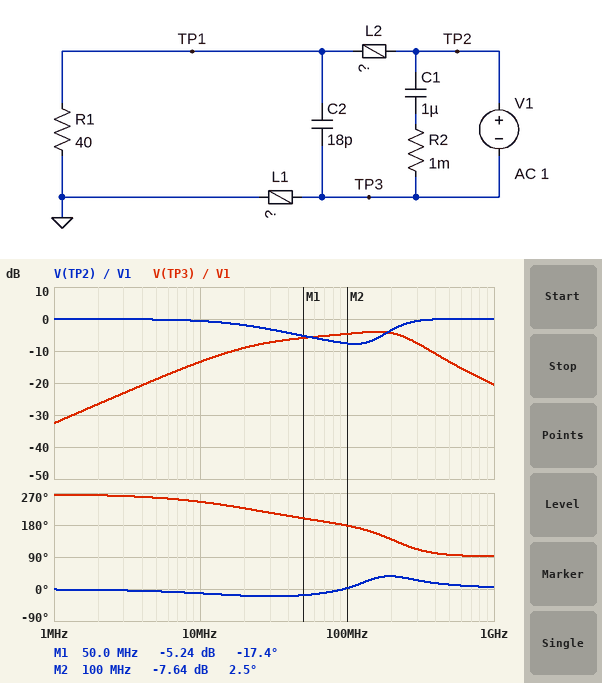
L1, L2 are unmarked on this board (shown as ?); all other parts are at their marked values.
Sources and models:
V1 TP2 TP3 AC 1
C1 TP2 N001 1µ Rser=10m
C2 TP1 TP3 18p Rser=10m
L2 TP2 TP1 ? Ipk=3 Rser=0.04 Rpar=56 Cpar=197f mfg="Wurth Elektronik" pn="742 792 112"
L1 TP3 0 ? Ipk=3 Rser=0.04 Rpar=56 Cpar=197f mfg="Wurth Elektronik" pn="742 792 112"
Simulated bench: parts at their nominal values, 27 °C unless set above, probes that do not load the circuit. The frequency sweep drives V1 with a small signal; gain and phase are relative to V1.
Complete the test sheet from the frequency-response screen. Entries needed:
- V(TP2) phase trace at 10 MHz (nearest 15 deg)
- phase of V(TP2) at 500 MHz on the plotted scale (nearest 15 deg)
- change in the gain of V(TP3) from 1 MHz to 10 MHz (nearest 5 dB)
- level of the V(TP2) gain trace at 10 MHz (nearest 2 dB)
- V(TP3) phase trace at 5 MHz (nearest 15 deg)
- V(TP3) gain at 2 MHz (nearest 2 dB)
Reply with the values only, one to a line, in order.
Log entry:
-15 deg
15 deg
20 dB
0 dB
255 deg
-26 dB
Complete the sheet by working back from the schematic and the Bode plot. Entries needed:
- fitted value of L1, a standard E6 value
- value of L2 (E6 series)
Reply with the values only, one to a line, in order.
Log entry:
150 nH
33 nH
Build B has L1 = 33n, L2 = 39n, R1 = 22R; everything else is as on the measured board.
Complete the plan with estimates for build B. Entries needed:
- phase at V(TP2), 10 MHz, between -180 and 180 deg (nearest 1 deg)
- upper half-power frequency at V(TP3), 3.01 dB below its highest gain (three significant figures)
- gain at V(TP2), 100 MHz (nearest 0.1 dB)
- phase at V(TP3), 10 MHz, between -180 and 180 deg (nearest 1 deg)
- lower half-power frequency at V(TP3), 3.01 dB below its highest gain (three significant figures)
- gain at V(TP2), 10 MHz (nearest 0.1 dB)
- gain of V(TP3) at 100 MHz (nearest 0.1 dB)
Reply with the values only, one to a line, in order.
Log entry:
-5 deg
371 MHz
-4.1 dB
-105 deg
69.7 MHz
-0.2 dB
-7.8 dB
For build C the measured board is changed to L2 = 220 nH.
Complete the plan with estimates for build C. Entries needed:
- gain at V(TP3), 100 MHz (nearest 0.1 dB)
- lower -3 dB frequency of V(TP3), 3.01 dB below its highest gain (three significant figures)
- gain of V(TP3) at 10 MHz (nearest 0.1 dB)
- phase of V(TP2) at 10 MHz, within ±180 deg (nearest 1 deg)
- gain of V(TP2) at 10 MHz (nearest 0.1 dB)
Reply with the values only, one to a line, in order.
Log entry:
-8.5 dB
19.6 MHz
-14.5 dB
-10 deg
-0.9 dB
